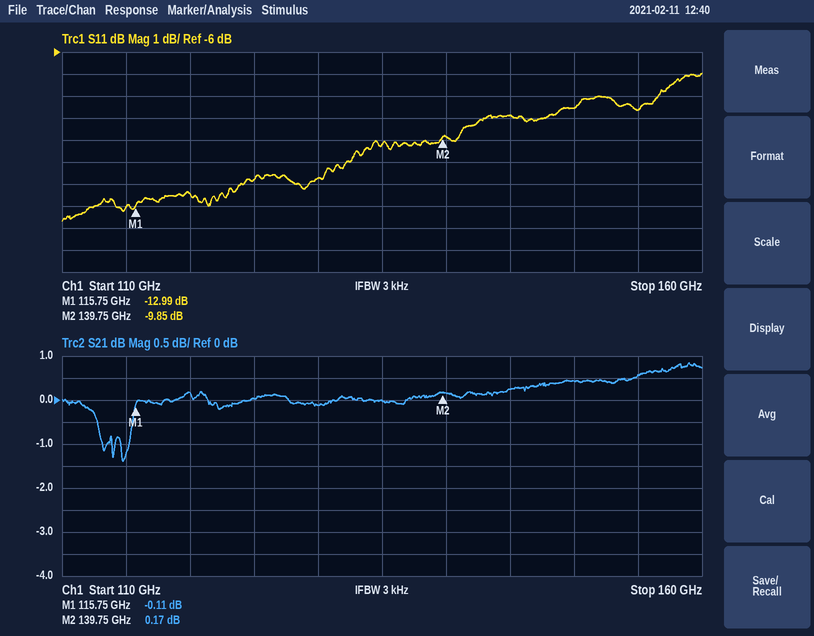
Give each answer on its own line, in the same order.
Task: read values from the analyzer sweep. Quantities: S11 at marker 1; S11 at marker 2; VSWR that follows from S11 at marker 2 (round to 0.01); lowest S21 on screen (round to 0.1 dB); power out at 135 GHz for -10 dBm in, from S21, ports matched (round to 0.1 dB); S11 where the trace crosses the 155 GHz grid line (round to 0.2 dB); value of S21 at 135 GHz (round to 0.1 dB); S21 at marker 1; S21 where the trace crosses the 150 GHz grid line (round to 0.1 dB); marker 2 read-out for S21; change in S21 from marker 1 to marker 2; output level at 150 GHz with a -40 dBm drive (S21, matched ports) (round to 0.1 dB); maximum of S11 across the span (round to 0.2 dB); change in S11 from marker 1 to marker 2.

-12.99 dB
-9.85 dB
1.95
-1.4 dB
-10.0 dBm
-8.6 dB
0.0 dB
-0.11 dB
0.4 dB
0.17 dB
0.28 dB
-39.6 dBm
-7.0 dB
3.14 dB
